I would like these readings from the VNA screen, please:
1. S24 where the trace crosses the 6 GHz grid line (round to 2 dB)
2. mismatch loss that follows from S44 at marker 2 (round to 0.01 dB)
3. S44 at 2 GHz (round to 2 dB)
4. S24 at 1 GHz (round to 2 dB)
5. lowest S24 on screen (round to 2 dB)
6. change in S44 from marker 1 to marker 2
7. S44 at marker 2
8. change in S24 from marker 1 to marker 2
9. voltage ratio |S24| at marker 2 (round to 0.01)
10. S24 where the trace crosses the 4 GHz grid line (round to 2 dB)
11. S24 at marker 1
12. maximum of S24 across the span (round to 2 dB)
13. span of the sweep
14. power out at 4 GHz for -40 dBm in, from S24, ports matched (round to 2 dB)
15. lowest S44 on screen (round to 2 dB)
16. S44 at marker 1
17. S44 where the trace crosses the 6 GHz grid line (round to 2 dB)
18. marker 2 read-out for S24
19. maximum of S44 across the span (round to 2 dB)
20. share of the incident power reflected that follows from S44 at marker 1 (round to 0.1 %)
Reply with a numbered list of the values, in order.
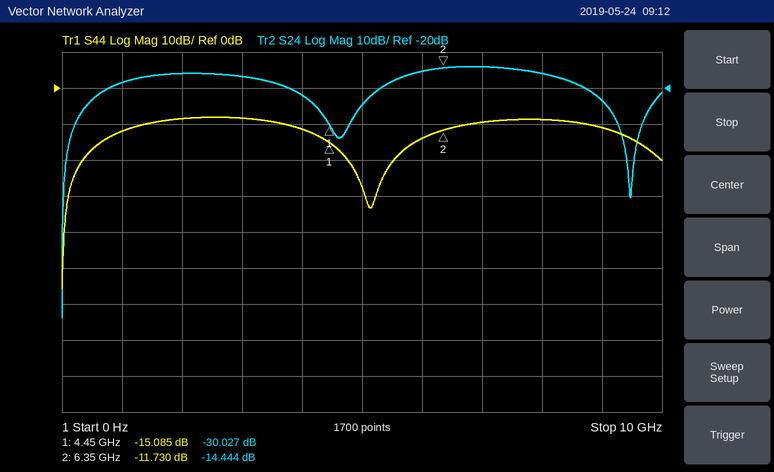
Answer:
1. -16 dB
2. 0.30 dB
3. -8 dB
4. -18 dB
5. -84 dB
6. 3.355 dB
7. -11.730 dB
8. 15.583 dB
9. 0.19
10. -22 dB
11. -30.027 dB
12. -14 dB
13. 10 GHz
14. -62 dBm
15. -56 dB
16. -15.085 dB
17. -14 dB
18. -14.444 dB
19. -8 dB
20. 3.1 %
